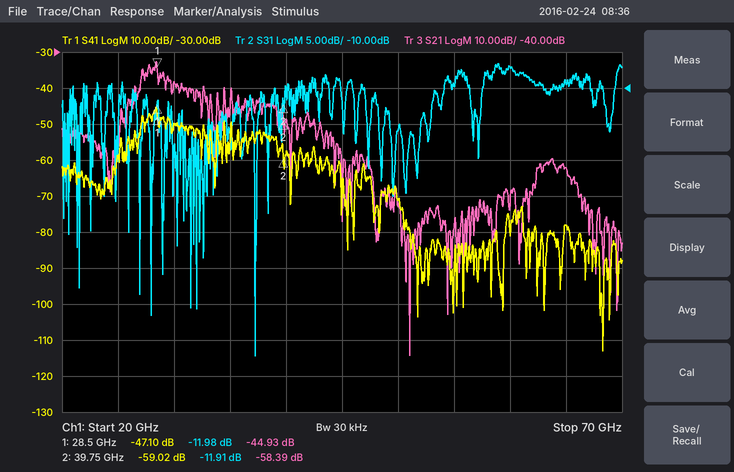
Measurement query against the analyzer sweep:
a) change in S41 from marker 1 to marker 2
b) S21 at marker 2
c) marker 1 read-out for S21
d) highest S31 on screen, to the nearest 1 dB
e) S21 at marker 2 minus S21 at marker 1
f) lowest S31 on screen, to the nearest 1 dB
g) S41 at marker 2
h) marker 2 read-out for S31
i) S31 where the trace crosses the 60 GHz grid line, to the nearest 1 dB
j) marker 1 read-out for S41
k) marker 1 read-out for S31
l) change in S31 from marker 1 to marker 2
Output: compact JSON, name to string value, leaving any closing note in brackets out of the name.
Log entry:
{"change in S41 from marker 1 to marker 2": "-11.92 dB", "S21 at marker 2": "-58.39 dB", "marker 1 read-out for S21": "-44.93 dB", "highest S31 on screen, to the nearest 1 dB": "-7 dB", "S21 at marker 2 minus S21 at marker 1": "-13.46 dB", "lowest S31 on screen, to the nearest 1 dB": "-47 dB", "S41 at marker 2": "-59.02 dB", "marker 2 read-out for S31": "-11.91 dB", "S31 where the trace crosses the 60 GHz grid line, to the nearest 1 dB": "-7 dB", "marker 1 read-out for S41": "-47.10 dB", "marker 1 read-out for S31": "-11.98 dB", "change in S31 from marker 1 to marker 2": "0.07 dB"}
